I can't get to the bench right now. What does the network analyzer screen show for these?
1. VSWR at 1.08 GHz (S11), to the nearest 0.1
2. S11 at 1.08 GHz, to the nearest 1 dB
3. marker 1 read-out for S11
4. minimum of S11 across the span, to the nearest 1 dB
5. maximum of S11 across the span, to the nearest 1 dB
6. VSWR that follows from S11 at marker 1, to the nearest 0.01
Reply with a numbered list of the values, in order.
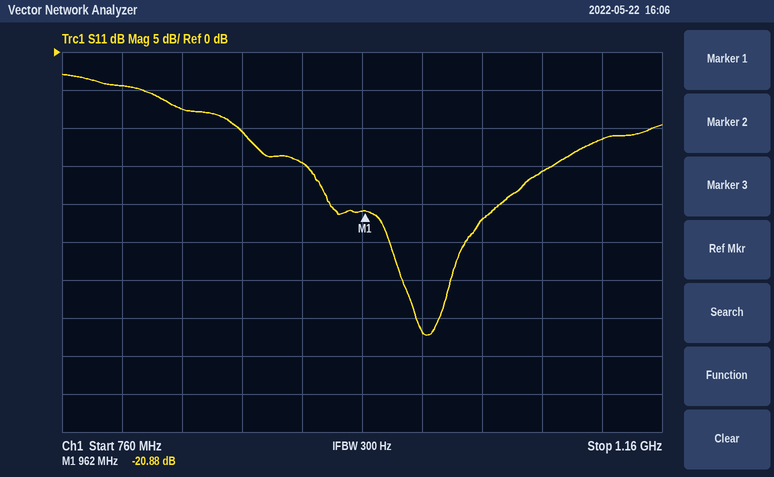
1. 1.4
2. -16 dB
3. -20.88 dB
4. -37 dB
5. -3 dB
6. 1.20
